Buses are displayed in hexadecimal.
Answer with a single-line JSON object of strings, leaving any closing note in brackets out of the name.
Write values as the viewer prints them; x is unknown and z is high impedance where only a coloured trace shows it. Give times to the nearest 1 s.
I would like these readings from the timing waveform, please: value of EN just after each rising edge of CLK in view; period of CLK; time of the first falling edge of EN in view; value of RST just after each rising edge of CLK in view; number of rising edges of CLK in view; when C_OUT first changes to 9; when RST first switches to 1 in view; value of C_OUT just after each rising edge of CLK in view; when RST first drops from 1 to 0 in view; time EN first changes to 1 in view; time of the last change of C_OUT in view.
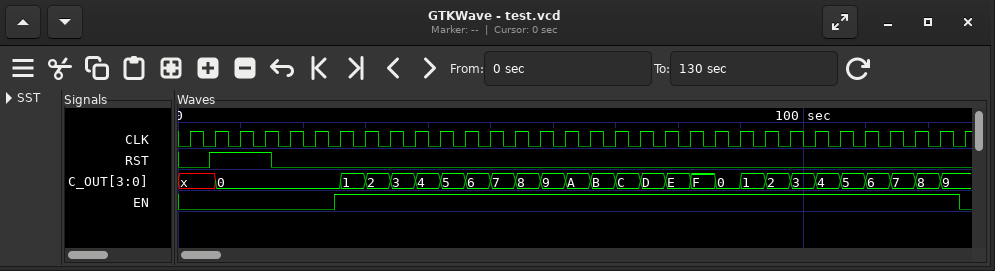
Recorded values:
{"value of EN just after each rising edge of CLK in view": "0 0 0 0 0 0 1 1 1 1 1 1 1 1 1 1 1 1 1 1 1 1 1 1 1 1 1 1 1 1 1 0", "period of CLK": "4 s", "time of the first falling edge of EN in view": "125 s", "value of RST just after each rising edge of CLK in view": "0 1 1 1 0 0 0 0 0 0 0 0 0 0 0 0 0 0 0 0 0 0 0 0 0 0 0 0 0 0 0 0", "number of rising edges of CLK in view": "32", "when C_OUT first changes to 9": "58 s", "when RST first switches to 1 in view": "5 s", "value of C_OUT just after each rising edge of CLK in view": "x, 0, 0, 0, 0, 0, 1, 2, 3, 4, 5, 6, 7, 8, 9, A, B, C, D, E, F, 0, 1, 2, 3, 4, 5, 6, 7, 8, 9, 9", "when RST first drops from 1 to 0 in view": "15 s", "time EN first changes to 1 in view": "25 s", "time of the last change of C_OUT in view": "122 s"}
